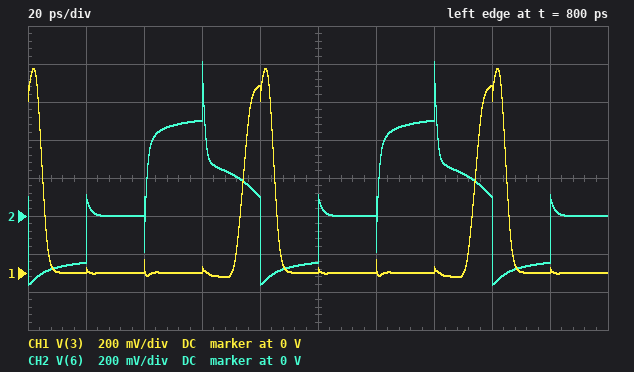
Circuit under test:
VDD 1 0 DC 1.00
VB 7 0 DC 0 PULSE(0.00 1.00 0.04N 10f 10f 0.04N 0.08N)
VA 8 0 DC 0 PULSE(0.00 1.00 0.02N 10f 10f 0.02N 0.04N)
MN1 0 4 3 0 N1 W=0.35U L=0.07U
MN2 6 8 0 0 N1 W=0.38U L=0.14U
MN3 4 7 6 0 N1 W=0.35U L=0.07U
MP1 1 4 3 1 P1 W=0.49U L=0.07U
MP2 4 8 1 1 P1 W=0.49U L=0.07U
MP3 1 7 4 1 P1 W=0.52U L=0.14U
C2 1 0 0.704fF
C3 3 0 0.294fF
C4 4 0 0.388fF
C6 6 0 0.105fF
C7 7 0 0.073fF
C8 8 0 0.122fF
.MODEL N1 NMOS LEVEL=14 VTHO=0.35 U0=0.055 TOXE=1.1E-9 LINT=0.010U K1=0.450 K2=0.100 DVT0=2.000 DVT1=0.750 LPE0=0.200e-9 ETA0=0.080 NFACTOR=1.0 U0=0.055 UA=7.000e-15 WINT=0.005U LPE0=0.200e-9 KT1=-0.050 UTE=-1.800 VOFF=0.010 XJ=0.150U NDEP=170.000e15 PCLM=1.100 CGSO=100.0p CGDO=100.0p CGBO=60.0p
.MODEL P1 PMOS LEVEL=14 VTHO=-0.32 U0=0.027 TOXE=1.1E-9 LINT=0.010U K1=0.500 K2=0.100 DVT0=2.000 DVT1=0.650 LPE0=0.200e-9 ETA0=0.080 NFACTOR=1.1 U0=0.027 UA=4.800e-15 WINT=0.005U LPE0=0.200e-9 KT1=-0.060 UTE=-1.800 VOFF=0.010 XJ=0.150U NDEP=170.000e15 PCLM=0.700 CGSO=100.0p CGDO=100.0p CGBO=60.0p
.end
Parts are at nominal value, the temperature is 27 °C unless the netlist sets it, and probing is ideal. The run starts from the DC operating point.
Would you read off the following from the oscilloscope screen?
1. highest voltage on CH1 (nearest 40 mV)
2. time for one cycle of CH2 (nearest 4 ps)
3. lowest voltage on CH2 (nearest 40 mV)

1.08 V
80 ps
-360 mV
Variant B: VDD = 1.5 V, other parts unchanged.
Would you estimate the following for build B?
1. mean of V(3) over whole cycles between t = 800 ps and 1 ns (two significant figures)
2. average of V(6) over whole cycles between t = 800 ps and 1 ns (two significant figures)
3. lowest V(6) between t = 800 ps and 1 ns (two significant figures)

57 mV
150 mV
-210 mV
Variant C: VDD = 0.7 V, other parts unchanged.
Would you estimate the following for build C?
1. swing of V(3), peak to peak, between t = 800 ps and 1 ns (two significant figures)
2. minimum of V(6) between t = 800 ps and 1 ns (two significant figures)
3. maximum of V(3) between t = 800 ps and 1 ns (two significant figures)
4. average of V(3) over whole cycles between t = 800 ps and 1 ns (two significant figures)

870 mV
-420 mV
800 mV
120 mV
